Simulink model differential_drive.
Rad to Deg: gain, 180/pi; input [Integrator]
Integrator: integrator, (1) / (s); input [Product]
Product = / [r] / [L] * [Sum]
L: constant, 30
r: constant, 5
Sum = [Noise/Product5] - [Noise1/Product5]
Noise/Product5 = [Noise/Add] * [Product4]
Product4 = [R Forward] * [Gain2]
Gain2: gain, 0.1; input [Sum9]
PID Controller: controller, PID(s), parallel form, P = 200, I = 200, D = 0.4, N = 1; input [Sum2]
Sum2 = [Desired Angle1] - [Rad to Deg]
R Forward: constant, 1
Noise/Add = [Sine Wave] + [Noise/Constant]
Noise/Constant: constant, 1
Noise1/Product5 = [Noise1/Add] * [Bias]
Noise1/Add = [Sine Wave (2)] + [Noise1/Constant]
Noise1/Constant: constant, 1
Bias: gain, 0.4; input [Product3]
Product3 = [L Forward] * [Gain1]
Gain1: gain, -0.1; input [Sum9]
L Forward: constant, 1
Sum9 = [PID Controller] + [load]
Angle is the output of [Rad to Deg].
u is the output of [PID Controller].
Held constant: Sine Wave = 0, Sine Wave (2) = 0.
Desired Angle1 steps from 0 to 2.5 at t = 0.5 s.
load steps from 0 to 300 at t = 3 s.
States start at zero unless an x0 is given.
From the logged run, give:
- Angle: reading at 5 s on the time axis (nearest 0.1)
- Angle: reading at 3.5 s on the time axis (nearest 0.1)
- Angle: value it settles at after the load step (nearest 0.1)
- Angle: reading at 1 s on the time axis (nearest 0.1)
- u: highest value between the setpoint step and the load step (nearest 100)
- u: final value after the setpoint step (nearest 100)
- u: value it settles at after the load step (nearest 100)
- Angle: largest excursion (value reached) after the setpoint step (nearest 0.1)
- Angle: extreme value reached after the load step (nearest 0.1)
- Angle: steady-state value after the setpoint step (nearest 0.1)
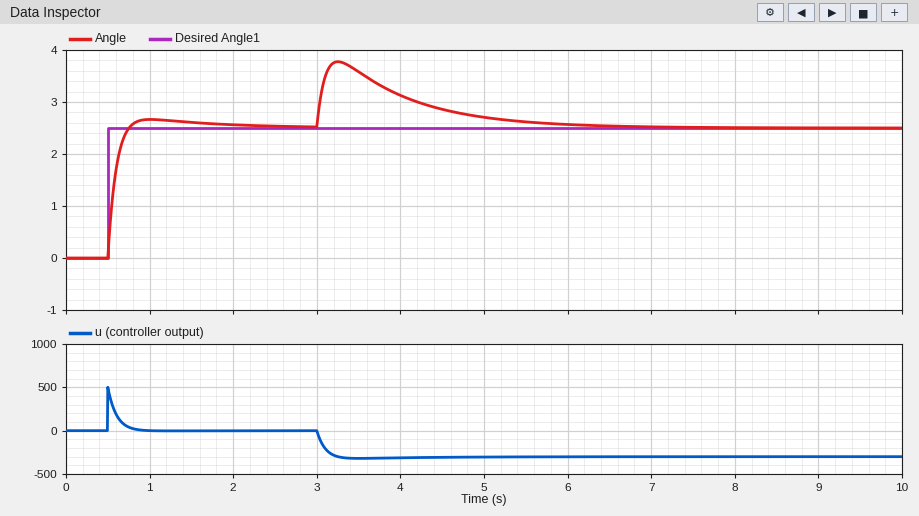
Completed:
2.7
3.6
2.5
2.7
500
0
-300
2.7
3.8
2.5
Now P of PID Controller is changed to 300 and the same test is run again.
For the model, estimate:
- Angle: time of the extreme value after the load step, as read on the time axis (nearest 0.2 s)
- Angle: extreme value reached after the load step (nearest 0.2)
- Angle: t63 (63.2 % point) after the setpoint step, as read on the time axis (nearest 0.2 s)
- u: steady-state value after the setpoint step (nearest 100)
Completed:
3.2 s
3.4
0.6 s
0
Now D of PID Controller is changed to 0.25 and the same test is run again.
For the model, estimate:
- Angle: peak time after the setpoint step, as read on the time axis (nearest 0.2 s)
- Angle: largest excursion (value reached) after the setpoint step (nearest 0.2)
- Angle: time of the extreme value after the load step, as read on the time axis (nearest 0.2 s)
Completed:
1.0 s
2.6
3.2 s
